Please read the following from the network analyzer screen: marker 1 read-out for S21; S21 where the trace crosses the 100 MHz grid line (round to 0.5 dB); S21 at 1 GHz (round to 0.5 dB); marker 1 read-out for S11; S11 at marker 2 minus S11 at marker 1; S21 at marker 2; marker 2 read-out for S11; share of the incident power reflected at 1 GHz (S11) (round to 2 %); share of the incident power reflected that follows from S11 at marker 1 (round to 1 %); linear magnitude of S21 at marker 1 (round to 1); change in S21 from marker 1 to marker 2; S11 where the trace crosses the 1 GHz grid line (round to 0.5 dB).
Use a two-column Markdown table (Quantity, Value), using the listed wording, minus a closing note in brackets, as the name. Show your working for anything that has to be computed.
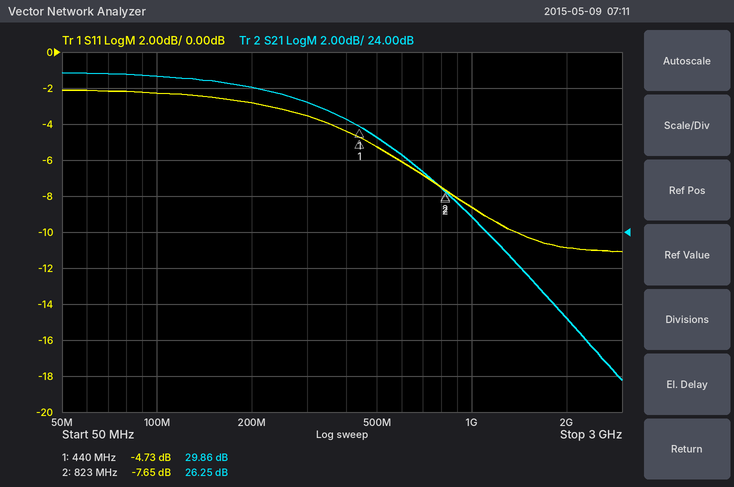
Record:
| Quantity | Value |
|---|---|
| marker 1 read-out for S21 | 29.86 dB |
| S21 where the trace crosses the 100 MHz grid line | 32.5 dB |
| S21 at 1 GHz | 25.0 dB |
| marker 1 read-out for S11 | -4.73 dB |
| S11 at marker 2 minus S11 at marker 1 | -7.65 − (-4.73) = -2.92 dB |
| S21 at marker 2 | 26.25 dB |
| marker 2 read-out for S11 | -7.65 dB |
| share of the incident power reflected at 1 GHz (S11) | 10^(-8.5/10) ≈ 14 % |
| share of the incident power reflected that follows from S11 at marker 1 | 10^(-4.73/10) ≈ 34 % |
| linear magnitude of S21 at marker 1 | 10^(29.86/20) ≈ 31 |
| change in S21 from marker 1 to marker 2 | 26.25 − (29.86) = -3.61 dB |
| S11 where the trace crosses the 1 GHz grid line | -8.5 dB |
